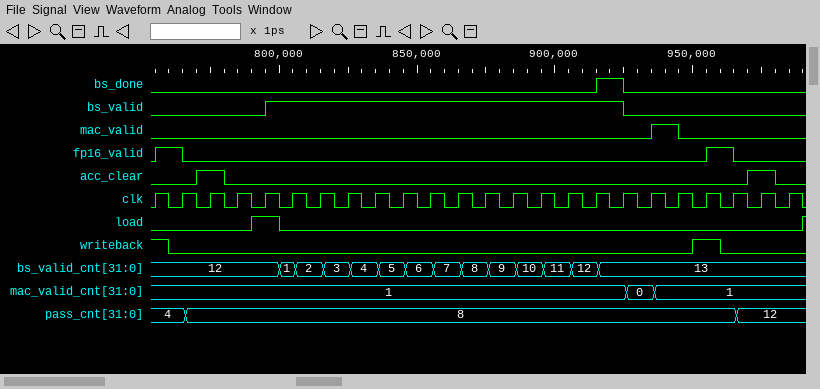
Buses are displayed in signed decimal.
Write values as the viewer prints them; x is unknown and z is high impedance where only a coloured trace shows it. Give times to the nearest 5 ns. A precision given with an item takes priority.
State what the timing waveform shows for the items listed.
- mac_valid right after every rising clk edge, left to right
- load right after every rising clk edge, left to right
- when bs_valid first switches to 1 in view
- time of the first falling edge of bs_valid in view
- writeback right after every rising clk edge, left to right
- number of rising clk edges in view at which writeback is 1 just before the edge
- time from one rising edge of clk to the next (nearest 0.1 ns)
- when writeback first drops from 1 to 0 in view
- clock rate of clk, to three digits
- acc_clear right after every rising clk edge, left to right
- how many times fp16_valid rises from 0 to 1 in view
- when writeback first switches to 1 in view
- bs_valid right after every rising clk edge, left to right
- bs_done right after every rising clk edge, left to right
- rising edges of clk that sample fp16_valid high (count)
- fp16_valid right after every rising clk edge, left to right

0 0 0 0 0 0 0 0 0 0 0 0 0 0 0 0 0 0 1 0 0 0 0 0
0 0 0 0 1 0 0 0 0 0 0 0 0 0 0 0 0 0 0 0 0 0 0 0
795 ns
925 ns
1 0 0 0 0 0 0 0 0 0 0 0 0 0 0 0 0 0 0 0 1 0 0 0
2
10 ns
760 ns
100 MHz
0 0 1 0 0 0 0 0 0 0 0 0 0 0 0 0 0 0 0 0 0 0 1 0
2
950 ns
0 0 0 0 1 1 1 1 1 1 1 1 1 1 1 1 1 0 0 0 0 0 0 0
0 0 0 0 0 0 0 0 0 0 0 0 0 0 0 0 1 0 0 0 0 0 0 0
2
1 0 0 0 0 0 0 0 0 0 0 0 0 0 0 0 0 0 0 0 1 0 0 0
